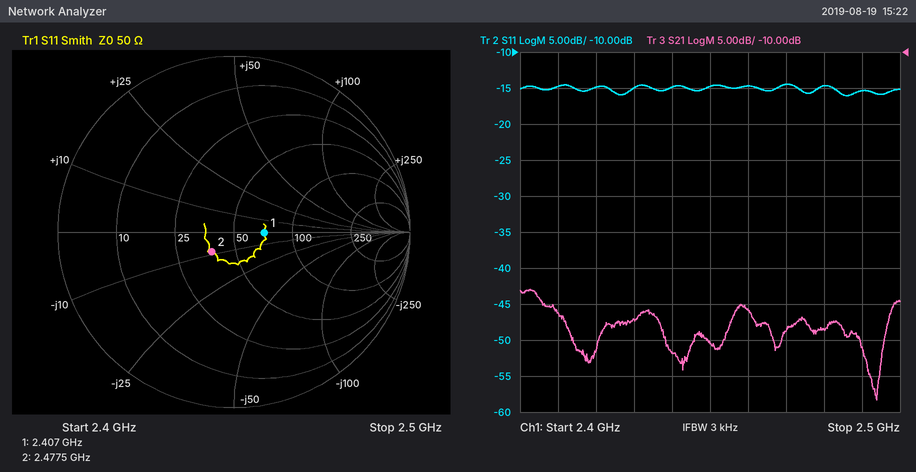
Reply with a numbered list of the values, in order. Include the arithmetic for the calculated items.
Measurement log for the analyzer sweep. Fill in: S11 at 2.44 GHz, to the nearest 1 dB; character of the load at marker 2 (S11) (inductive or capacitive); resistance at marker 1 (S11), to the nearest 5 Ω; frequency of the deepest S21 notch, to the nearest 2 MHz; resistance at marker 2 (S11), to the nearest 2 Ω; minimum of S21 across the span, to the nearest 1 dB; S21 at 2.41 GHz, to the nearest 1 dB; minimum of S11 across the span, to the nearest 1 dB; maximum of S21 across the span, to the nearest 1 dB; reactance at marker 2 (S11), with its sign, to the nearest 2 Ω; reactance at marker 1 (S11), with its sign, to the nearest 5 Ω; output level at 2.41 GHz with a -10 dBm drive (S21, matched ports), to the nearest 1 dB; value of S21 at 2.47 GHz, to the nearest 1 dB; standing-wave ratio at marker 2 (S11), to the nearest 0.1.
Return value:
1. -15 dB
2. capacitive
3. 70 Ω
4. 2.494 GHz
5. 38 Ω
6. -58 dB
7. -46 dB
8. -16 dB
9. -43 dB
10. -8 Ω
11. 0 Ω
12. -10 dBm + (-46 dB) = -56 dBm
13. -49 dB
14. 1.4
